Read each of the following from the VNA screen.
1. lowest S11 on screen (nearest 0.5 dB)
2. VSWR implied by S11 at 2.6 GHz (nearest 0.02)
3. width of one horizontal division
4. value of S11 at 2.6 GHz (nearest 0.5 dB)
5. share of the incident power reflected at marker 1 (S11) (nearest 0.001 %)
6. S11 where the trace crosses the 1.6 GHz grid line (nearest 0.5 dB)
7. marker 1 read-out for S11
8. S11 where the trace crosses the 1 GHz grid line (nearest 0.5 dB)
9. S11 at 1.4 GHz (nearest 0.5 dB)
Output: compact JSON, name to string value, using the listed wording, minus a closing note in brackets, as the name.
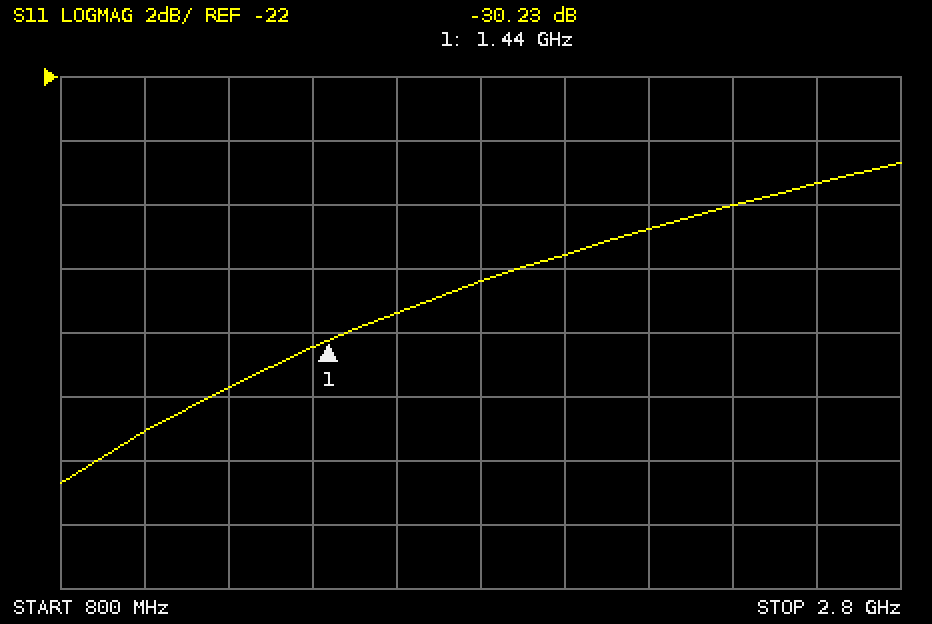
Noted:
{"lowest S11 on screen": "-34.5 dB", "VSWR implied by S11 at 2.6 GHz": "1.12", "width of one horizontal division": "200 MHz", "value of S11 at 2.6 GHz": "-25.5 dB", "share of the incident power reflected at marker 1 (S11)": "0.095 %", "S11 where the trace crosses the 1.6 GHz grid line": "-29.5 dB", "marker 1 read-out for S11": "-30.23 dB", "S11 where the trace crosses the 1 GHz grid line": "-33.0 dB", "S11 at 1.4 GHz": "-30.5 dB"}
